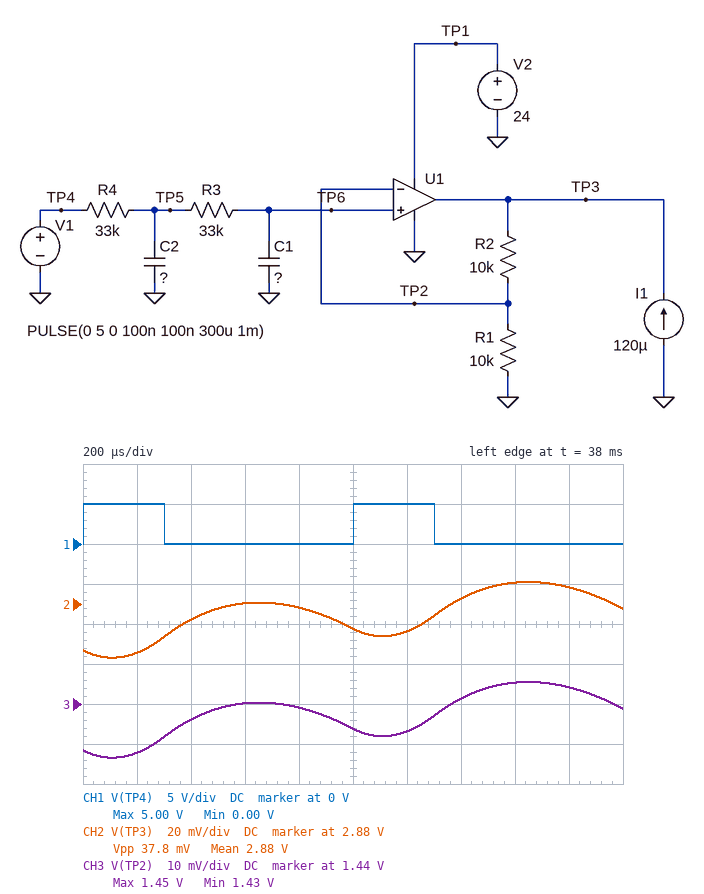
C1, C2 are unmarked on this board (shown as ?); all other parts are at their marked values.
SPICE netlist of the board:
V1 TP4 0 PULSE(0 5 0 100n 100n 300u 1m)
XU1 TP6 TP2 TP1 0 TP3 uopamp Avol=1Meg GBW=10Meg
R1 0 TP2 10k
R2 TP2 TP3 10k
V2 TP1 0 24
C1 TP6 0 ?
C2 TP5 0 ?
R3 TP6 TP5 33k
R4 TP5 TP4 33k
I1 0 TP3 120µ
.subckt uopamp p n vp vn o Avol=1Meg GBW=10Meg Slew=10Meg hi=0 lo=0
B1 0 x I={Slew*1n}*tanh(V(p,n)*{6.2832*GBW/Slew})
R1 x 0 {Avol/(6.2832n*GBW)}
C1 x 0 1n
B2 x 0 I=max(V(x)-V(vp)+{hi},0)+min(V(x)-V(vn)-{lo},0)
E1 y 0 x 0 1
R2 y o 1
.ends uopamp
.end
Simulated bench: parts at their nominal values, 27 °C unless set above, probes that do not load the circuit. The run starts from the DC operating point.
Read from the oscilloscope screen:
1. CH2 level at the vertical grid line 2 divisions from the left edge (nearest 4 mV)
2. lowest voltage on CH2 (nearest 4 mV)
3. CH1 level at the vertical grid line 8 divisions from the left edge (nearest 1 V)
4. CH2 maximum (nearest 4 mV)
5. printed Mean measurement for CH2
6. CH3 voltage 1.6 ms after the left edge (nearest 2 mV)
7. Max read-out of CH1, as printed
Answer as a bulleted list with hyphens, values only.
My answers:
- 2.872 V
- 2.852 V
- 0 V
- 2.892 V
- 2.88 V
- 1.446 V
- 5.00 V
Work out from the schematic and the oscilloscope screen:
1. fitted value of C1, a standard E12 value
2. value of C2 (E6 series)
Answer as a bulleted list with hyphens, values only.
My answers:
- 33 nF
- 330 nF
